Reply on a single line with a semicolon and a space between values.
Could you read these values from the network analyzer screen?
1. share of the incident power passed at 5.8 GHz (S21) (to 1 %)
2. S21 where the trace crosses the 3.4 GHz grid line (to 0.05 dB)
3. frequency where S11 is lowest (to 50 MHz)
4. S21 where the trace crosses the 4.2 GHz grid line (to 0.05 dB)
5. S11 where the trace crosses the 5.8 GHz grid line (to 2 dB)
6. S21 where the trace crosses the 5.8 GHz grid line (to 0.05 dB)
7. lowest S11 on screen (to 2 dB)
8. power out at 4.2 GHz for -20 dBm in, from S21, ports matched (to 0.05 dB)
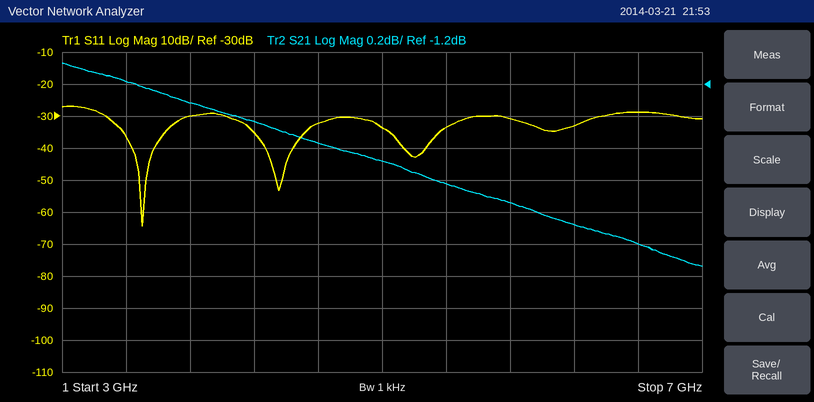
64 %; -1.20 dB; 3.50 GHz; -1.45 dB; -30 dB; -1.95 dB; -64 dB; -21.45 dBm
